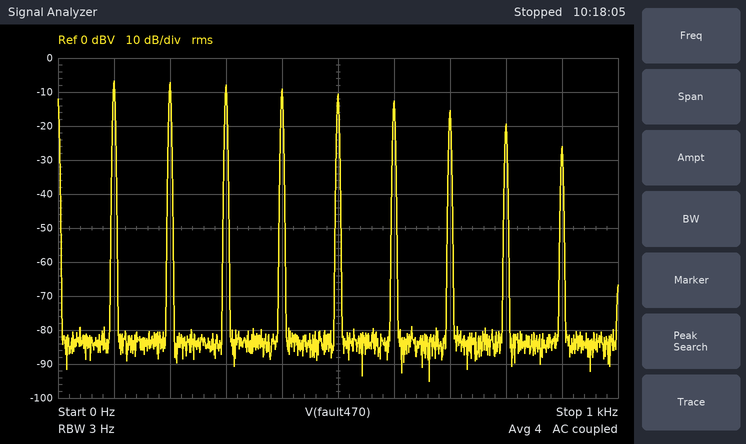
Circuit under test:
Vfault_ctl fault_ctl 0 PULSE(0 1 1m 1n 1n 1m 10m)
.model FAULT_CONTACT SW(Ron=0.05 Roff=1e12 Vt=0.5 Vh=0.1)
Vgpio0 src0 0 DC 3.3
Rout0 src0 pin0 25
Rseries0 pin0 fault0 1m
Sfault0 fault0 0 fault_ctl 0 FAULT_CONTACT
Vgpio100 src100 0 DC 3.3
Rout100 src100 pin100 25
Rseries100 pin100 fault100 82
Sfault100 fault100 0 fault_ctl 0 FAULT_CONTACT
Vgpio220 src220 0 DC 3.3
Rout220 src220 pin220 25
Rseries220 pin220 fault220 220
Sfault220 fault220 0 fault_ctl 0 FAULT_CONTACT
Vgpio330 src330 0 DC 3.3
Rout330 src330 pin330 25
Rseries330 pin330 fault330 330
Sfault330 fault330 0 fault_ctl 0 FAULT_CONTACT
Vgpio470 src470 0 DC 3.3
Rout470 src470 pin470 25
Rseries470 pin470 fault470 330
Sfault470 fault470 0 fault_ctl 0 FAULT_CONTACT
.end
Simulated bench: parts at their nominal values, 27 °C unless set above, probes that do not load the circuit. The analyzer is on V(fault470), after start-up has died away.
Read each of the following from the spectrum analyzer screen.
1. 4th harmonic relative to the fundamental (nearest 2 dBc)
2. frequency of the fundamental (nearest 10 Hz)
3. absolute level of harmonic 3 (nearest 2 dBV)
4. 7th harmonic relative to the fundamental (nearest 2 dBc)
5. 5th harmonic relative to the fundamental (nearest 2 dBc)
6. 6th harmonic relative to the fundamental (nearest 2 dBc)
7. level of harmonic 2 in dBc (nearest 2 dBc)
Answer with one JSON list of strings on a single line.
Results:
["-2 dBc", "100 Hz", "-8 dBV", "-8 dBc", "-4 dBc", "-6 dBc", "0 dBc"]
